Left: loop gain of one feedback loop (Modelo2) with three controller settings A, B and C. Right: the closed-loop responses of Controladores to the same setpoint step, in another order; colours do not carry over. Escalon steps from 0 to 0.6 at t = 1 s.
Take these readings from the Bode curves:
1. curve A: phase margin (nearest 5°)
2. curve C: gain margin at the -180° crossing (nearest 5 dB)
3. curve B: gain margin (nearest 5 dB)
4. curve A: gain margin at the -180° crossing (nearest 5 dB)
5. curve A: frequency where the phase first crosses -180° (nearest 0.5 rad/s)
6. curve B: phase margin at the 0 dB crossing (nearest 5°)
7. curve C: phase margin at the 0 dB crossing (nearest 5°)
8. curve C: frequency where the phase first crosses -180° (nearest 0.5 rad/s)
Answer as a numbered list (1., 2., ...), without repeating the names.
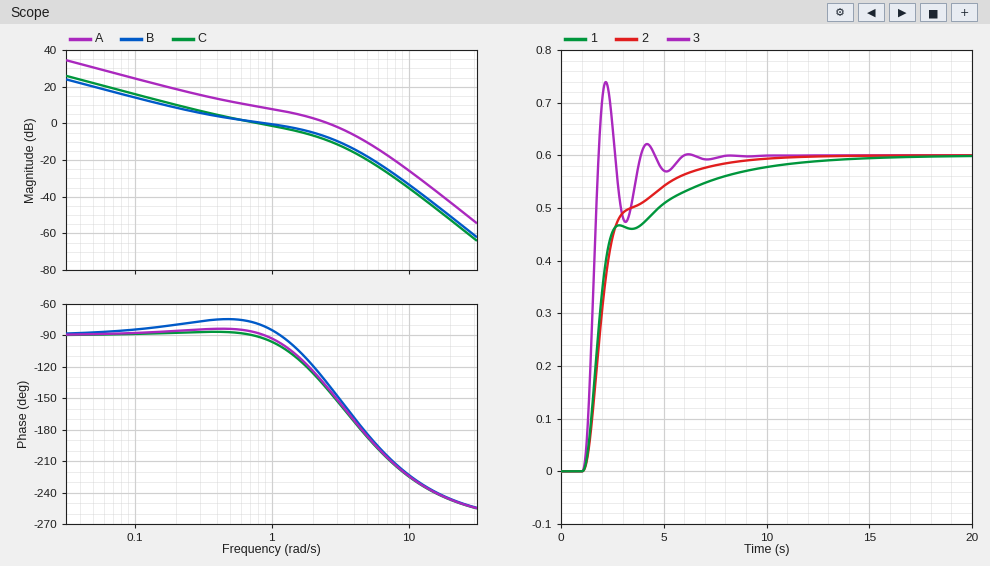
1. 40°
2. 20 dB
3. 15 dB
4. 10 dB
5. 4.5 rad/s
6. 100°
7. 90°
8. 4.5 rad/s
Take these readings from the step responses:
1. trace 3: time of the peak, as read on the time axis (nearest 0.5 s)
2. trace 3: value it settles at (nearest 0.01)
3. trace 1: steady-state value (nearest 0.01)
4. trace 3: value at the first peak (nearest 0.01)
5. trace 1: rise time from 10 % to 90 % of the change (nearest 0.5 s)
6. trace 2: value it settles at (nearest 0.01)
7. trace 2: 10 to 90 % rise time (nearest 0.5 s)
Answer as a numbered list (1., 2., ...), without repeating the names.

1. 2.0 s
2. 0.60
3. 0.60
4. 0.74
5. 5.0 s
6. 0.60
7. 3.5 s
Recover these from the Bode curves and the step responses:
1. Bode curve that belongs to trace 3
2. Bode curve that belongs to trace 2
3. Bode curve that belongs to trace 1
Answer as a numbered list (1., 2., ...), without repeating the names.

1. A
2. C
3. B
